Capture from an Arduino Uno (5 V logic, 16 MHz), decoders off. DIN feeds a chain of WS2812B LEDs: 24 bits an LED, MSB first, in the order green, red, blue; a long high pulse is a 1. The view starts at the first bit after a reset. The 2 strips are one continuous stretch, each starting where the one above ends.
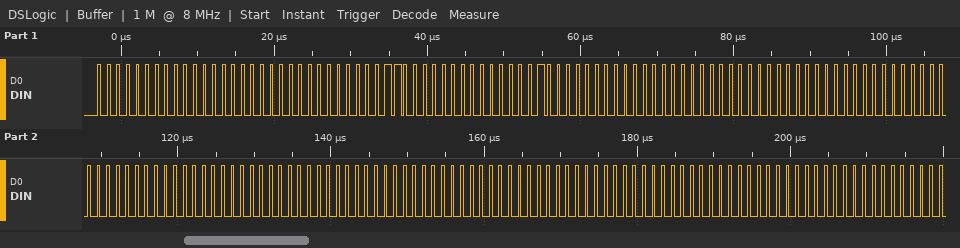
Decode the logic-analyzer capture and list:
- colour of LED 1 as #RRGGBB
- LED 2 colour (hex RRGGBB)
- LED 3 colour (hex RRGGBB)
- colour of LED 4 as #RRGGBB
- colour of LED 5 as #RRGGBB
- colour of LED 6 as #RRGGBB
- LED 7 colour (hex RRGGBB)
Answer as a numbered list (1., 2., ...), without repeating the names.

1. #000000
2. #000302
3. #000000
4. #000000
5. #000000
6. #000000
7. #000000
